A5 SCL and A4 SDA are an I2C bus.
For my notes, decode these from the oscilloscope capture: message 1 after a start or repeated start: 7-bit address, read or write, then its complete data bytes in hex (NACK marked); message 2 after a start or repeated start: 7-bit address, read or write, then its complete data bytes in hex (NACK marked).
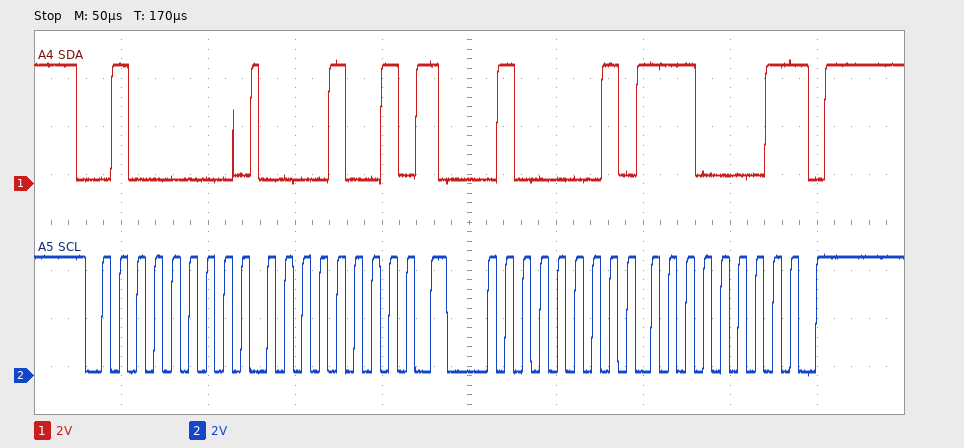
0x20 write: 09
0x20 read: E1 NACK
